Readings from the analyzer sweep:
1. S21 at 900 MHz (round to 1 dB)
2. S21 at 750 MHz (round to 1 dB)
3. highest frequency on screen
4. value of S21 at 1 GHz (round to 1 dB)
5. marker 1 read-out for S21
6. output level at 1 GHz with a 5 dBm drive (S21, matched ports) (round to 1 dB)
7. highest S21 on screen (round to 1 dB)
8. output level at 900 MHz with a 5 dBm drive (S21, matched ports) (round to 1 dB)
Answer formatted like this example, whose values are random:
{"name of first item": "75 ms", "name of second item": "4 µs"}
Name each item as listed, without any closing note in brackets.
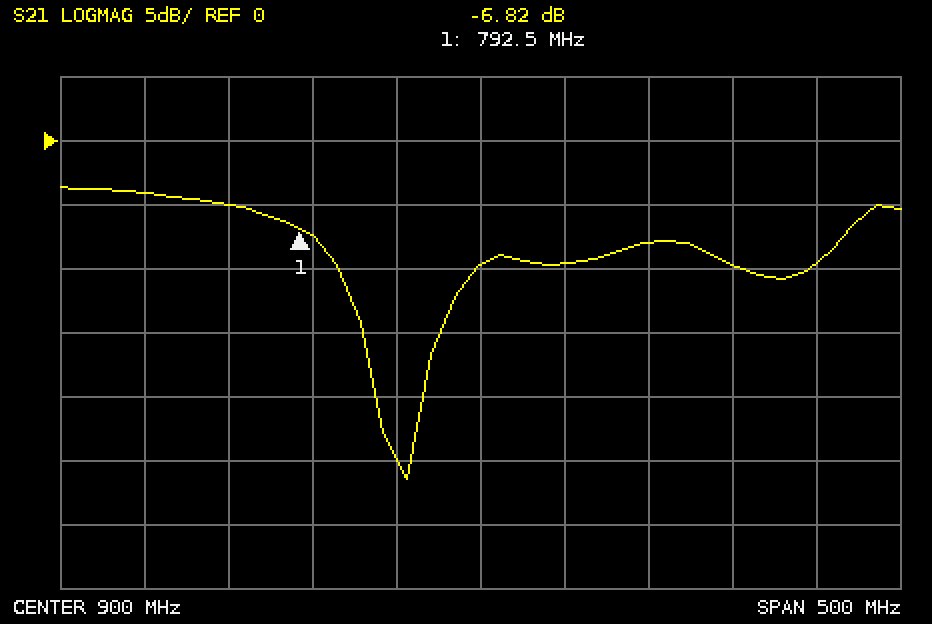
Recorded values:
{"S21 at 900 MHz": "-10 dB", "S21 at 750 MHz": "-5 dB", "highest frequency on screen": "1.15 GHz", "value of S21 at 1 GHz": "-8 dB", "marker 1 read-out for S21": "-6.82 dB", "output level at 1 GHz with a 5 dBm drive (S21, matched ports)": "-3 dBm", "highest S21 on screen": "-4 dB", "output level at 900 MHz with a 5 dBm drive (S21, matched ports)": "-5 dBm"}
